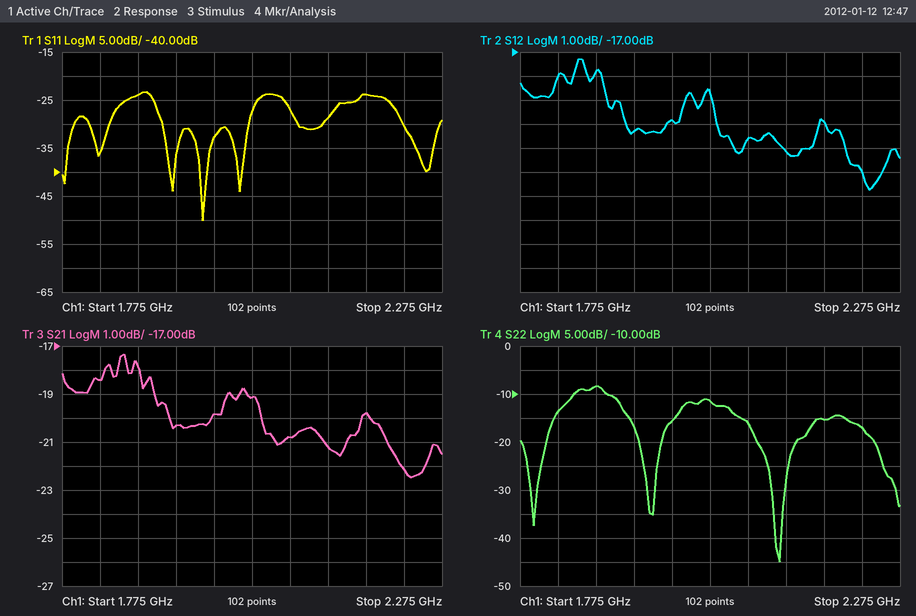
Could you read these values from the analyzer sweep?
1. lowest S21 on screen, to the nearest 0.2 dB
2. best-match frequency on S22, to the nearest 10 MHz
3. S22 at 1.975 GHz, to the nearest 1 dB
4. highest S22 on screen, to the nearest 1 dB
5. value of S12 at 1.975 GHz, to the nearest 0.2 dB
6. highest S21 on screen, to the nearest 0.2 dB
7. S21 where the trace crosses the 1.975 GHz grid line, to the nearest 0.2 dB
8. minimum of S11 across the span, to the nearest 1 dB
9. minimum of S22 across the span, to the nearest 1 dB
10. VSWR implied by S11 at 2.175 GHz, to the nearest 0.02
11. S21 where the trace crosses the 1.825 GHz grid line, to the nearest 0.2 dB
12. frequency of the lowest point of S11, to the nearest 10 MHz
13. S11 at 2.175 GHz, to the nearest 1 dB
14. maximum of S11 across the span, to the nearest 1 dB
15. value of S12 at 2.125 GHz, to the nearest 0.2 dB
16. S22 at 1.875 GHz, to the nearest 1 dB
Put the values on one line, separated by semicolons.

-22.4 dB; 2.12 GHz; -16 dB; -8 dB; -19.8 dB; -17.4 dB; -19.8 dB; -50 dB; -45 dB; 1.14; -18.4 dB; 1.96 GHz; -24 dB; -23 dB; -21.2 dB; -8 dB
